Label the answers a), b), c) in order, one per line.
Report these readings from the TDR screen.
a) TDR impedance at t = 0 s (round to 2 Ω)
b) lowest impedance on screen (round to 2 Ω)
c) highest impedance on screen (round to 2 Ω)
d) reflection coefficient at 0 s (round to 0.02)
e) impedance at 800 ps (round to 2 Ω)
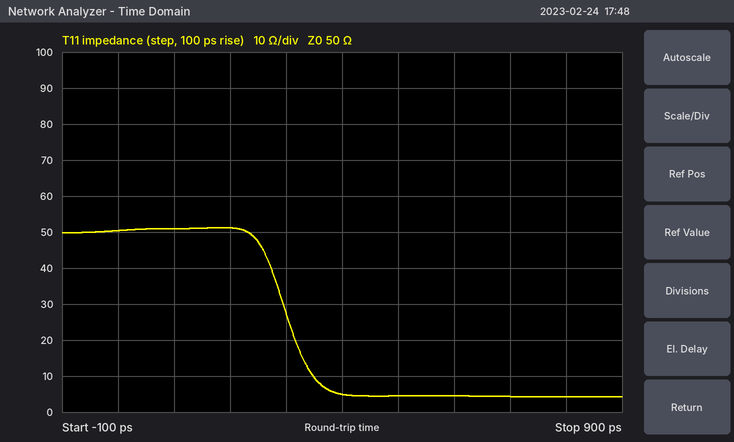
a) 50 Ω
b) 4 Ω
c) 52 Ω
d) 0.00
e) 4 Ω
